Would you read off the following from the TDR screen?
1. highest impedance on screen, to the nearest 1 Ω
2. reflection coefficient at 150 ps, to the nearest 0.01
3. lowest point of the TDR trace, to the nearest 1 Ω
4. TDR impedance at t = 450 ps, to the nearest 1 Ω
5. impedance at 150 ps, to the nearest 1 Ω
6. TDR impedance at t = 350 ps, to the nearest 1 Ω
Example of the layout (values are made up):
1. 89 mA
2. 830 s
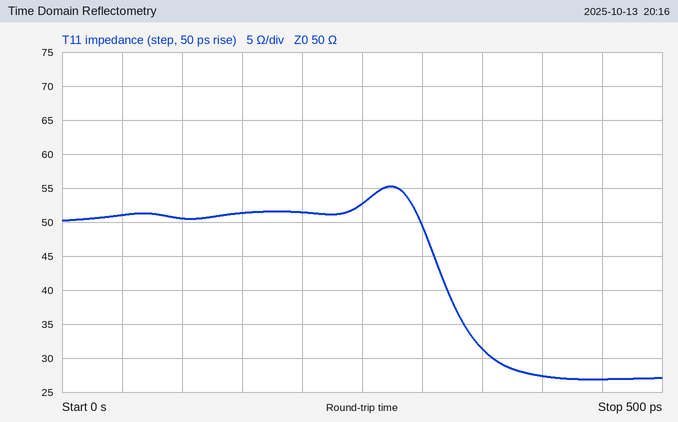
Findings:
1. 55 Ω
2. +0.01
3. 27 Ω
4. 27 Ω
5. 51 Ω
6. 31 Ω
